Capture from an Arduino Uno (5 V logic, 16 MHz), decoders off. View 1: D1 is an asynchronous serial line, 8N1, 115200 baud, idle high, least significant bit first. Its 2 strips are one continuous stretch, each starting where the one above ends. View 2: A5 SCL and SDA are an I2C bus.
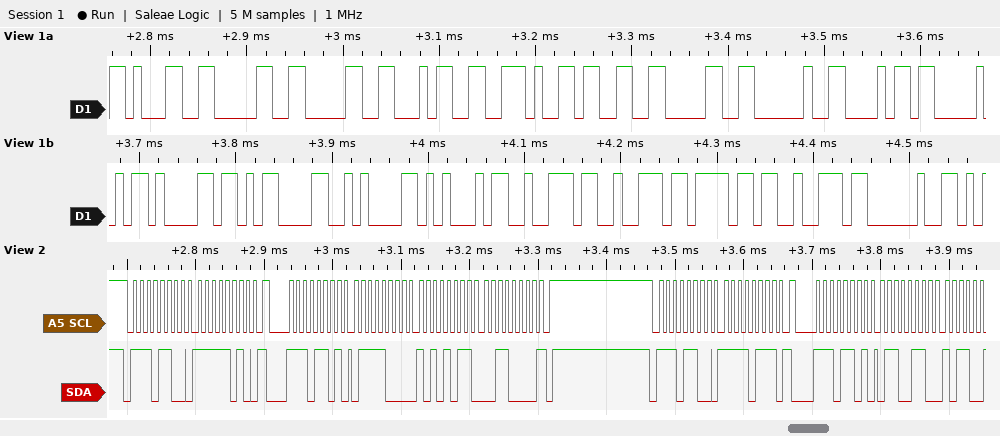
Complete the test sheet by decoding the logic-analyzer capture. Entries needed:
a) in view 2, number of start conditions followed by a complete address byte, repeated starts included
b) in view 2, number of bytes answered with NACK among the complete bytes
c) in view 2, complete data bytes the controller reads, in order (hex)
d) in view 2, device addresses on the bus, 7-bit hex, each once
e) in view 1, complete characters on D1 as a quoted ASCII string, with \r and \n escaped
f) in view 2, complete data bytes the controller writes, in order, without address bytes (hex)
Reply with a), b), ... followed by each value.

a) 4
b) 1
c) 78 AB 30 66
d) 0x76
e) "1004.30 hPa\r\nError "
f) FA F7
